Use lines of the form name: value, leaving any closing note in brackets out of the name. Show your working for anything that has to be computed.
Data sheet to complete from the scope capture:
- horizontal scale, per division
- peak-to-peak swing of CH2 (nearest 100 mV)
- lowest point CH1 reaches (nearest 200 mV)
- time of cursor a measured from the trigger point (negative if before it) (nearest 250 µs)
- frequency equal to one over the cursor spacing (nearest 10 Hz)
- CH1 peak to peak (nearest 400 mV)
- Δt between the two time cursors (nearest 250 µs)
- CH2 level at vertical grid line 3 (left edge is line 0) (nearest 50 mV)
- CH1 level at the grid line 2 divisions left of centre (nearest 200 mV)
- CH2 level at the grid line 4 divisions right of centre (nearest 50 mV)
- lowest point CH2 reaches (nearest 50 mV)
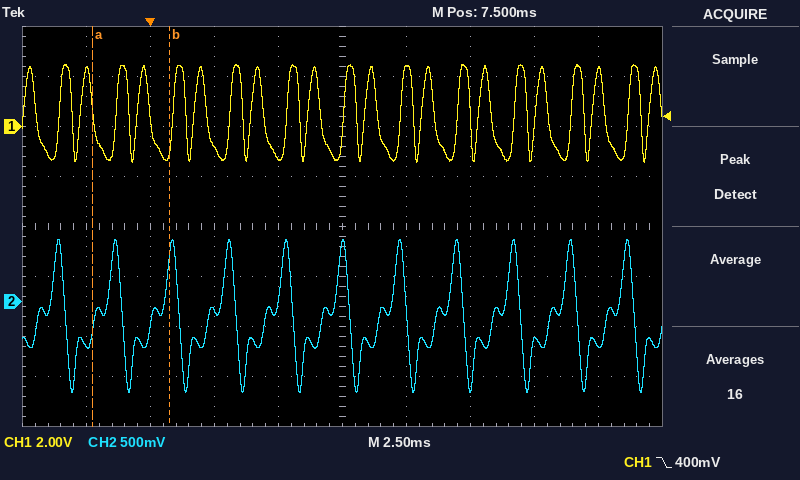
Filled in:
horizontal scale, per division: 2.5 ms
peak-to-peak swing of CH2: 1.50 V
lowest point CH1 reaches: -1.4 V
time of cursor a measured from the trigger point (negative if before it): -2.25 ms
frequency equal to one over the cursor spacing: 1 / 3.00 ms ≈ 330 Hz
CH1 peak to peak: 4.0 V
Δt between the two time cursors: 3.00 ms
CH2 level at vertical grid line 3 (left edge is line 0): -100 mV
CH1 level at the grid line 2 divisions left of centre: -800 mV
CH2 level at the grid line 4 divisions right of centre: -450 mV
lowest point CH2 reaches: -900 mV
